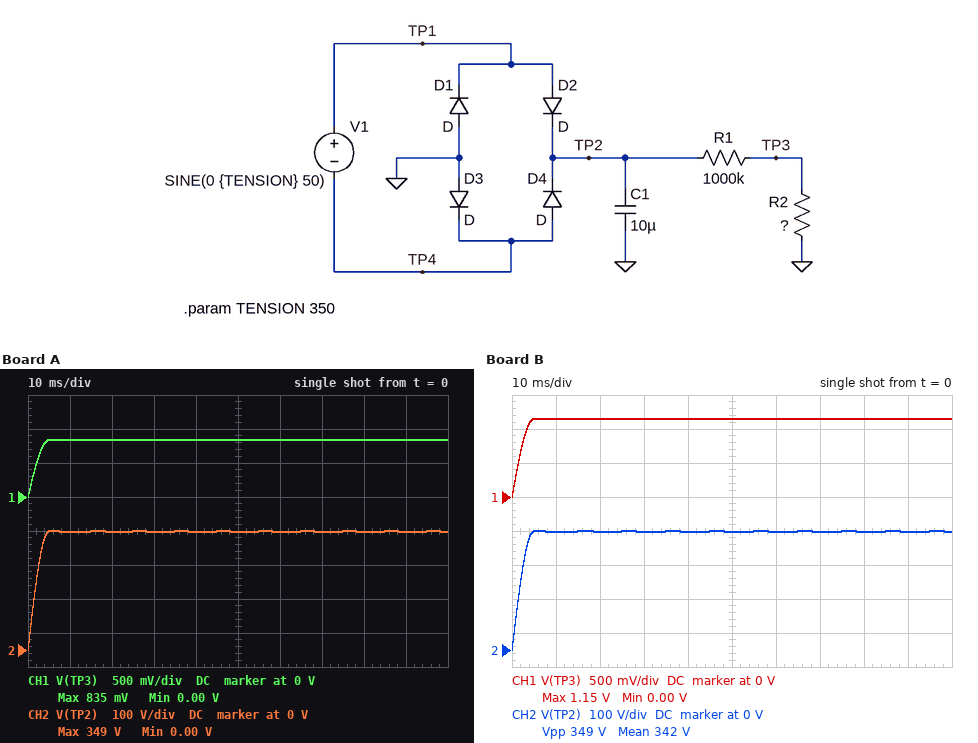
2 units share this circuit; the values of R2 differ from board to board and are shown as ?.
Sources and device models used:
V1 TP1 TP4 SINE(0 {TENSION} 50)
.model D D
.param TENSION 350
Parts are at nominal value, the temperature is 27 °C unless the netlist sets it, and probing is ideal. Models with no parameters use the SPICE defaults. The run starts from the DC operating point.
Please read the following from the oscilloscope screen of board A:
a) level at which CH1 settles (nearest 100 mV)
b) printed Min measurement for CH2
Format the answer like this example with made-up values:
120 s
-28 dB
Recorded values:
800 mV
0.00 V
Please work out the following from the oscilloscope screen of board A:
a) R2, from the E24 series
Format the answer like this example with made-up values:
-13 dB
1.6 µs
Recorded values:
2.4 kΩ
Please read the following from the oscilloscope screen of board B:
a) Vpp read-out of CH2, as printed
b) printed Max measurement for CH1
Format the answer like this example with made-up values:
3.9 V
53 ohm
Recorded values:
349 V
1.15 V
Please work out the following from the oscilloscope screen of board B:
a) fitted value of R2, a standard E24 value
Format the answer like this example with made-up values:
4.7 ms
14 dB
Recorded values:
3.3 kΩ
